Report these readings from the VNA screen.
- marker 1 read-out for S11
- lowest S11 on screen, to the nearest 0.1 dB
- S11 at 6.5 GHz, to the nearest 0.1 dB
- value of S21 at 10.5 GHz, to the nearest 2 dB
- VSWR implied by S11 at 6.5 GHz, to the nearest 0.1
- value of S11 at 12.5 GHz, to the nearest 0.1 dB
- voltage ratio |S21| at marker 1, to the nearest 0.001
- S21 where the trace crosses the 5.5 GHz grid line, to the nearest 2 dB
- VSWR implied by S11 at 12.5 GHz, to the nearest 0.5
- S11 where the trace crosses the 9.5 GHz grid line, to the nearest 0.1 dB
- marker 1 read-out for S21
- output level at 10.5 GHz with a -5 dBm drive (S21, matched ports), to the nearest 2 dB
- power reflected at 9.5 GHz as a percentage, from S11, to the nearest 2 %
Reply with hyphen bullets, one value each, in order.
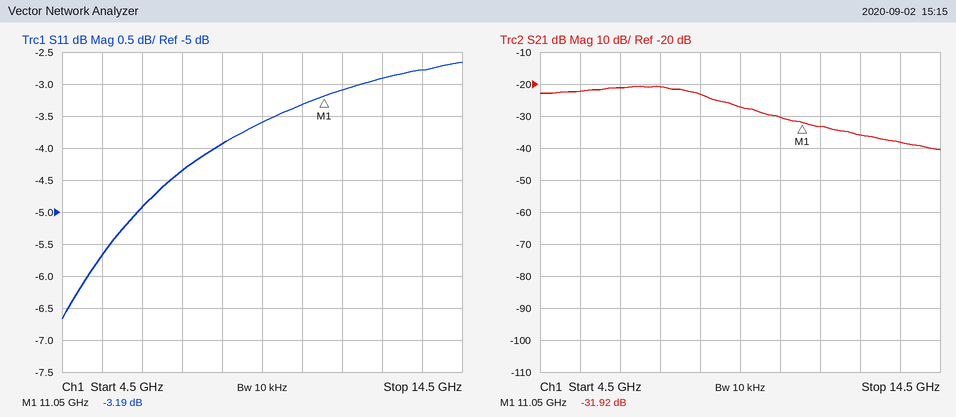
- -3.19 dB
- -6.7 dB
- -4.9 dB
- -30 dB
- 3.6
- -2.9 dB
- 0.025
- -22 dB
- 6.0
- -3.6 dB
- -31.92 dB
- -36 dBm
- 44 %
